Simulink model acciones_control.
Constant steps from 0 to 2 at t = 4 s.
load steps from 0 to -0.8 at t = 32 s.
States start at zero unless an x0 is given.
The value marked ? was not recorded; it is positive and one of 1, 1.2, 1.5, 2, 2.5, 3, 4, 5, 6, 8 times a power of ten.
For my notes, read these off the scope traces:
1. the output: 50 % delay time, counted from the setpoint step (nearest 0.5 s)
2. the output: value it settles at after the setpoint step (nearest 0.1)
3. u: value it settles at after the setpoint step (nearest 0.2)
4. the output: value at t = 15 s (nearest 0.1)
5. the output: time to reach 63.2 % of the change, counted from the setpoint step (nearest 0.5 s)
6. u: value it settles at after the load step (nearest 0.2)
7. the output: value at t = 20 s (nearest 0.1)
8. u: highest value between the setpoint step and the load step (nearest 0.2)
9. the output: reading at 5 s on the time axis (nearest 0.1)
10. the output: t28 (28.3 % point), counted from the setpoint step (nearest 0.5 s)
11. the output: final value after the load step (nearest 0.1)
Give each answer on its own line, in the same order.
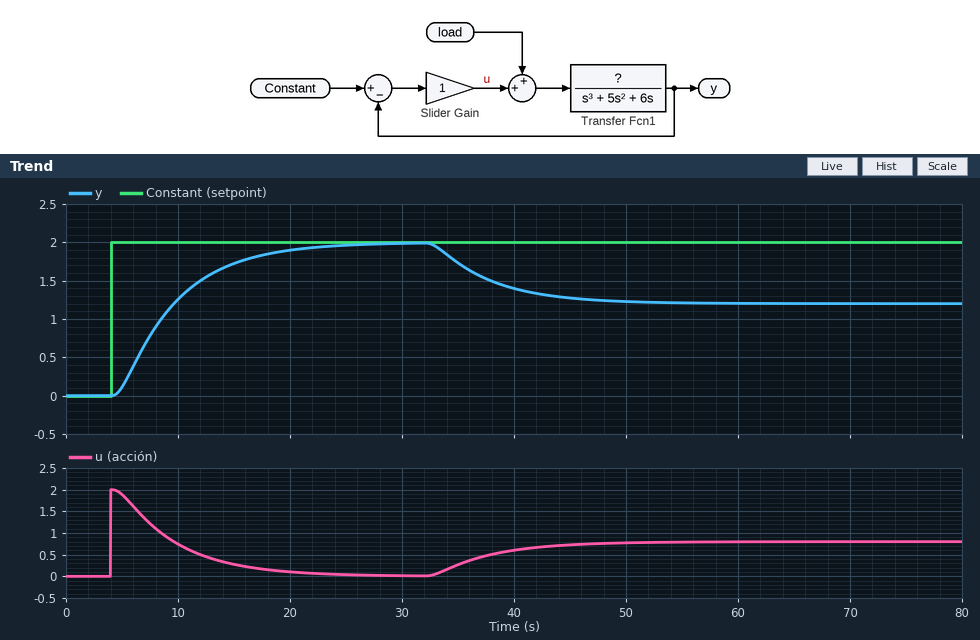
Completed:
4.5 s
2.0
0.0
1.7
6.0 s
0.8
1.9
2.0
0.1
2.5 s
1.2
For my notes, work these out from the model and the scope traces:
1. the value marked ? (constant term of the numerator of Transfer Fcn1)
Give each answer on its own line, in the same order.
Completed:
1
